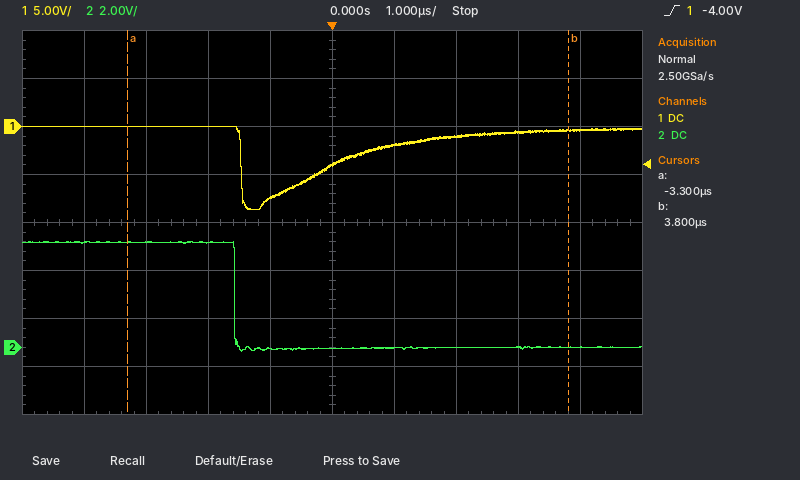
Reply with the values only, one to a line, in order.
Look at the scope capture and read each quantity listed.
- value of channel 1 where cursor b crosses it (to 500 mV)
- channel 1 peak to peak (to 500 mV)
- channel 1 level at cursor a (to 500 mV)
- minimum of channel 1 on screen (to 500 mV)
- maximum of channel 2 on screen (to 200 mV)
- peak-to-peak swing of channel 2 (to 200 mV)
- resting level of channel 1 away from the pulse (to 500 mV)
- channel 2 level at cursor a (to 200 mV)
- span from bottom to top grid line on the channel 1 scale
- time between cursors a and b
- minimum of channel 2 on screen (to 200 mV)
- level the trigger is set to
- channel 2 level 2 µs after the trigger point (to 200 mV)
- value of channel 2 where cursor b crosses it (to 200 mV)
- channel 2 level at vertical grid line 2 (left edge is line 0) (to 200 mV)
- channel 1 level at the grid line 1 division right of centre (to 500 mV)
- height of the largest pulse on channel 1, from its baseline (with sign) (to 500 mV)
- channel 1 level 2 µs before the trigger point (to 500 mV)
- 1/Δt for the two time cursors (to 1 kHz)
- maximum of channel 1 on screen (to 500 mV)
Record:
-500 mV
8.5 V
0.0 V
-8.5 V
4.4 V
4.6 V
0.0 V
4.4 V
40 V
7.1 µs
-200 mV
-4.00 V
0.0 V
0.0 V
4.4 V
-2.0 V
-8.5 V
0.0 V
141 kHz
0.0 V
